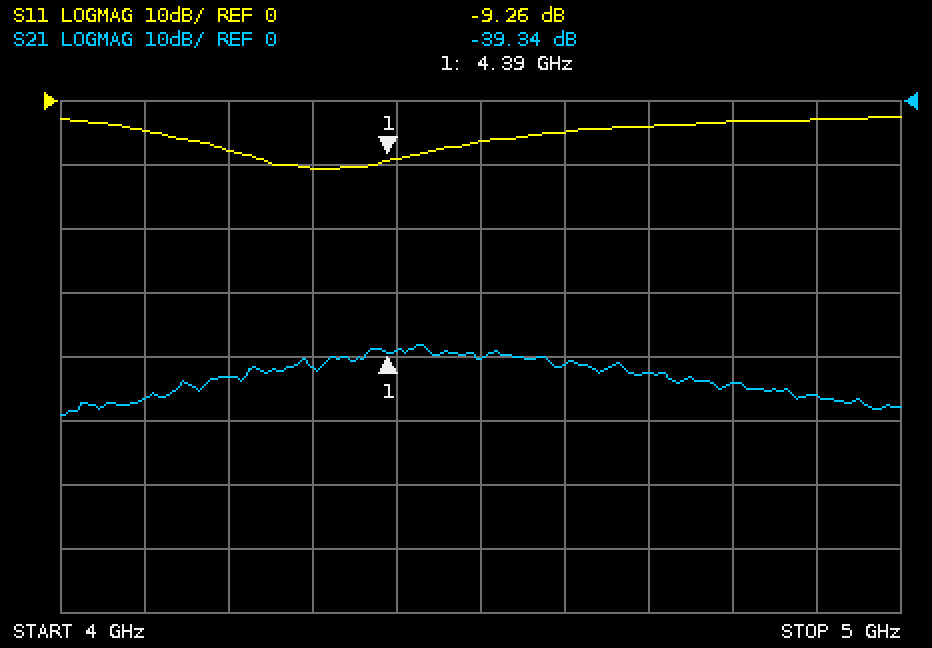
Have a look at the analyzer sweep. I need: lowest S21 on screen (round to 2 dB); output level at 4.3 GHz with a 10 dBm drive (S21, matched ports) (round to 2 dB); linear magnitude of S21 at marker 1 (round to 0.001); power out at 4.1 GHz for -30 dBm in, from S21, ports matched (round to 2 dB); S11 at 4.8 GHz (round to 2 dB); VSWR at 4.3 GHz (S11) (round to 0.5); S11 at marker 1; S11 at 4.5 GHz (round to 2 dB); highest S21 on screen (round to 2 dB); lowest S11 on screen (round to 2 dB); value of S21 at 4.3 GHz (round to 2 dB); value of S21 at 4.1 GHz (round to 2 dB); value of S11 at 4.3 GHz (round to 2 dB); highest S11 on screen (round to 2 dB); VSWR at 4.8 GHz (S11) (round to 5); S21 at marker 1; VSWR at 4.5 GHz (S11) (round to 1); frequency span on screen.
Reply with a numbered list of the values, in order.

1. -50 dB
2. -32 dBm
3. 0.011
4. -76 dBm
5. -4 dB
6. 2.0
7. -9.26 dB
8. -6 dB
9. -38 dB
10. -10 dB
11. -42 dB
12. -46 dB
13. -10 dB
14. -2 dB
15. 5
16. -39.34 dB
17. 3
18. 1 GHz
